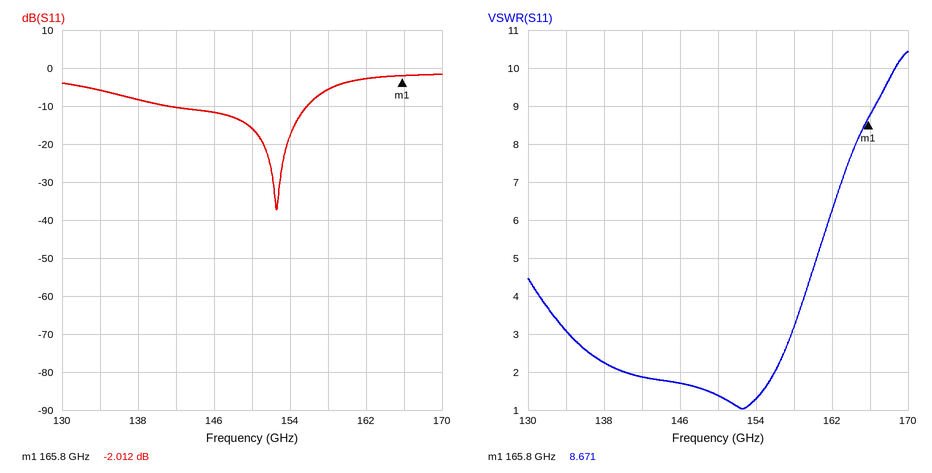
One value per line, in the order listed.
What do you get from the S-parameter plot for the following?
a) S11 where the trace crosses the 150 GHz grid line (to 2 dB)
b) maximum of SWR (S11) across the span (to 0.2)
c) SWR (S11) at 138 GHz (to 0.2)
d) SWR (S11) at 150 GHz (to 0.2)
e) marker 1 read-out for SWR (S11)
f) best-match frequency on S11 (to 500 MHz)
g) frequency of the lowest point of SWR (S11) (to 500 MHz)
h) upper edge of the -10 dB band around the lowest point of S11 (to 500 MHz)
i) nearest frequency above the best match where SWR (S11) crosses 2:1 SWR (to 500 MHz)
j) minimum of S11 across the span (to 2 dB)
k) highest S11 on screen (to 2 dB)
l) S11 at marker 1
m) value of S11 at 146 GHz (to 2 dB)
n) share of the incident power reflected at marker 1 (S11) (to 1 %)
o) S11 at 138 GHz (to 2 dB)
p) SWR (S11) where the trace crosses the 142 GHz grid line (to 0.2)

-16 dB
10.4
2.2
1.4
8.671
152.5 GHz
152.5 GHz
156.0 GHz
156.0 GHz
-38 dB
-2 dB
-2.012 dB
-12 dB
63 %
-8 dB
1.8
